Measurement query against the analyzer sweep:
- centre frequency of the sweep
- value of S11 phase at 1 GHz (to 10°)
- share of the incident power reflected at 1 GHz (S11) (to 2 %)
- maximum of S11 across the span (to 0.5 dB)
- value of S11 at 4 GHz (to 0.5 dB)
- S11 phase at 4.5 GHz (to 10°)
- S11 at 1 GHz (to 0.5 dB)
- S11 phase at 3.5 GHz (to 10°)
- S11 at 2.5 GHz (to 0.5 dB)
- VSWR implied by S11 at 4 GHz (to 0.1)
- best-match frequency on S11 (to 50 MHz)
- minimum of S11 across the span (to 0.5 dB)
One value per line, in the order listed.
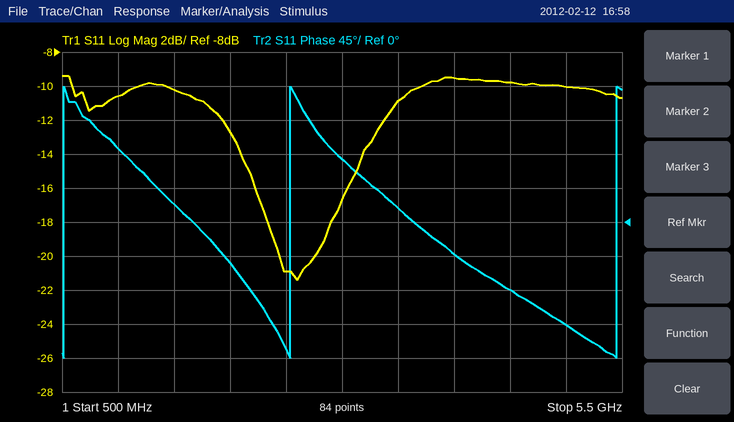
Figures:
3 GHz
100°
8 %
-9.5 dB
-9.5 dB
-90°
-10.5 dB
20°
-21.0 dB
2.0
2.60 GHz
-21.5 dB
